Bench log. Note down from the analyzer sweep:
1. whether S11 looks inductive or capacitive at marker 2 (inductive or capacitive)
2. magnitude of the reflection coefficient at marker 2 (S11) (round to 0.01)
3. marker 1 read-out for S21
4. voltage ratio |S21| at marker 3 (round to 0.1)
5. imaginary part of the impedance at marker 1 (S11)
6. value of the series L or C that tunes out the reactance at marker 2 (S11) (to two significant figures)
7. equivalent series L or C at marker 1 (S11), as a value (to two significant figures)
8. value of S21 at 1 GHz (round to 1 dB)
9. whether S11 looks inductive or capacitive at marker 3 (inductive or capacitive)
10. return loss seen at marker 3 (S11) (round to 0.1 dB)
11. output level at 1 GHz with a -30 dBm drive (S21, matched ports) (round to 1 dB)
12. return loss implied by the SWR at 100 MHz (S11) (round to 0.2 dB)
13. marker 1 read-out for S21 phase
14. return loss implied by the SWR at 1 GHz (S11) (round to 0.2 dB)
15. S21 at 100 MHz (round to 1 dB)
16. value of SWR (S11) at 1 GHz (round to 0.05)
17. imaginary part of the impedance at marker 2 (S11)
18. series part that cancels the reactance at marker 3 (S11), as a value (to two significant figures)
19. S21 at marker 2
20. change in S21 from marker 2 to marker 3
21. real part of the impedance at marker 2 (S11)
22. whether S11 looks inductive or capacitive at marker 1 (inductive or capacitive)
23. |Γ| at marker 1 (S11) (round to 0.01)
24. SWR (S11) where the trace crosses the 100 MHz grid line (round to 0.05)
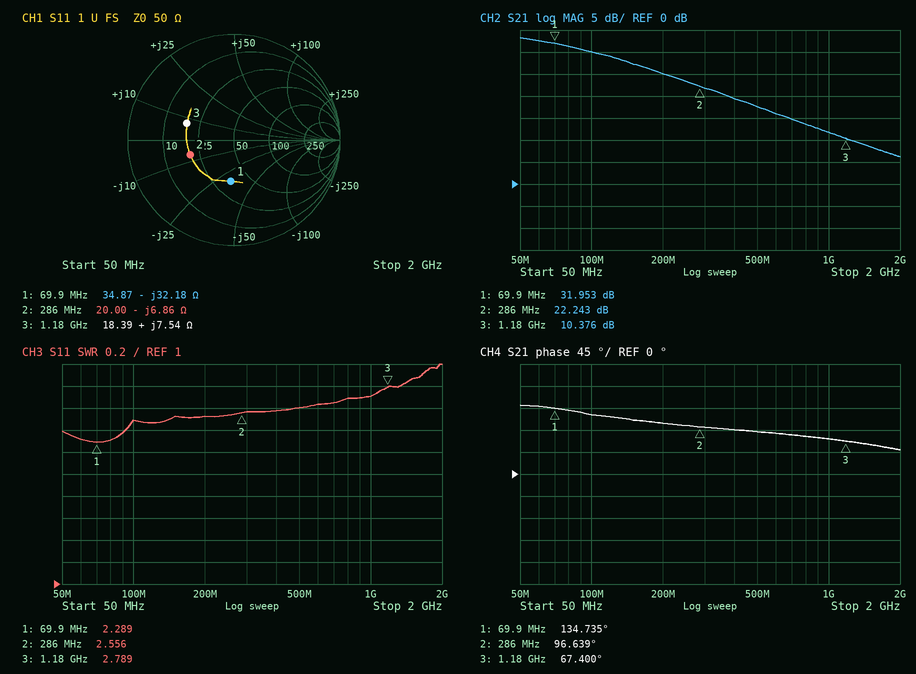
capacitive
0.44
31.953 dB
3.3
-32.18 Ω
3.8 nH
71 pF
12 dB
inductive
6.5 dB
-18 dBm
7.4 dB
134.735°
6.8 dB
30 dB
2.70
-6.86 Ω
18 pF
22.243 dB
-11.867 dB
20.00 Ω
capacitive
0.39
2.50
